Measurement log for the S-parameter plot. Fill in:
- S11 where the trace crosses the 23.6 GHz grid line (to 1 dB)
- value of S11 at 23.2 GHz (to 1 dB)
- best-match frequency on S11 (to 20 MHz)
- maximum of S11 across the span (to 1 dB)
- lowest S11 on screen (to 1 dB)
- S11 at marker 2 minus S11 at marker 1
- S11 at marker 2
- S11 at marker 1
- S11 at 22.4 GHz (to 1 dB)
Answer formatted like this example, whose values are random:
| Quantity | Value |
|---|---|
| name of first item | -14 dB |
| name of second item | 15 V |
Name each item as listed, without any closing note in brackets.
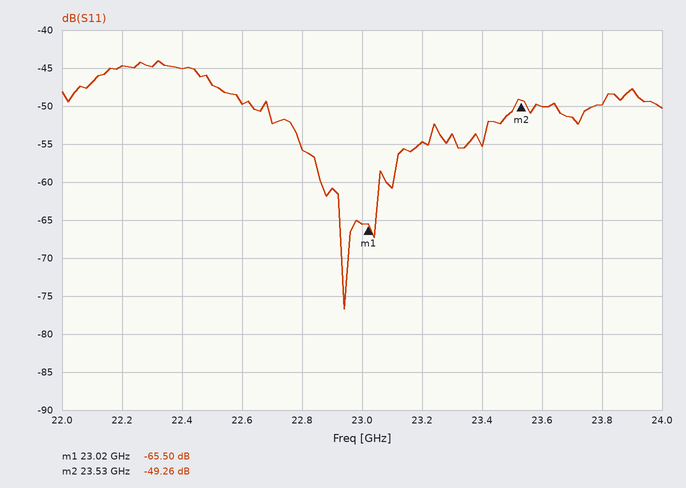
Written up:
| Quantity | Value |
|---|---|
| S11 where the trace crosses the 23.6 GHz grid line | -50 dB |
| value of S11 at 23.2 GHz | -55 dB |
| best-match frequency on S11 | 22.94 GHz |
| maximum of S11 across the span | -44 dB |
| lowest S11 on screen | -77 dB |
| S11 at marker 2 minus S11 at marker 1 | 16.24 dB |
| S11 at marker 2 | -49.26 dB |
| S11 at marker 1 | -65.50 dB |
| S11 at 22.4 GHz | -45 dB |
